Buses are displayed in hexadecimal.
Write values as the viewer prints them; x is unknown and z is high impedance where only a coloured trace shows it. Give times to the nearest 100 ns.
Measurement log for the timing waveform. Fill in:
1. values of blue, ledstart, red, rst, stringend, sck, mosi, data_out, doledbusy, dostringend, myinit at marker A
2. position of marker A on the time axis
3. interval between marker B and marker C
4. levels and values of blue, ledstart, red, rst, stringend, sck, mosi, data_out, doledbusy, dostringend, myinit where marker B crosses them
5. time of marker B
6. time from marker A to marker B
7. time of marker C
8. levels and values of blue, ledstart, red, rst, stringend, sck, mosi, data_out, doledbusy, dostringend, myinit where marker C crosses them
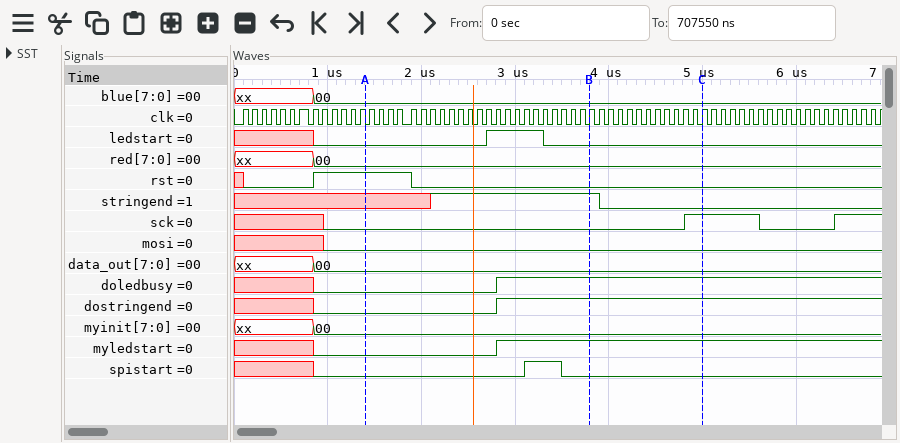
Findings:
blue=00, ledstart=0, red=00, rst=1, stringend=x, sck=0, mosi=0, data_out=00, doledbusy=0, dostringend=0, myinit=00
1400 ns
1200 ns
blue=00, ledstart=0, red=00, rst=0, stringend=1, sck=0, mosi=0, data_out=00, doledbusy=1, dostringend=1, myinit=00
3800 ns
2400 ns
5000 ns
blue=00, ledstart=0, red=00, rst=0, stringend=0, sck=1, mosi=0, data_out=00, doledbusy=1, dostringend=1, myinit=00
